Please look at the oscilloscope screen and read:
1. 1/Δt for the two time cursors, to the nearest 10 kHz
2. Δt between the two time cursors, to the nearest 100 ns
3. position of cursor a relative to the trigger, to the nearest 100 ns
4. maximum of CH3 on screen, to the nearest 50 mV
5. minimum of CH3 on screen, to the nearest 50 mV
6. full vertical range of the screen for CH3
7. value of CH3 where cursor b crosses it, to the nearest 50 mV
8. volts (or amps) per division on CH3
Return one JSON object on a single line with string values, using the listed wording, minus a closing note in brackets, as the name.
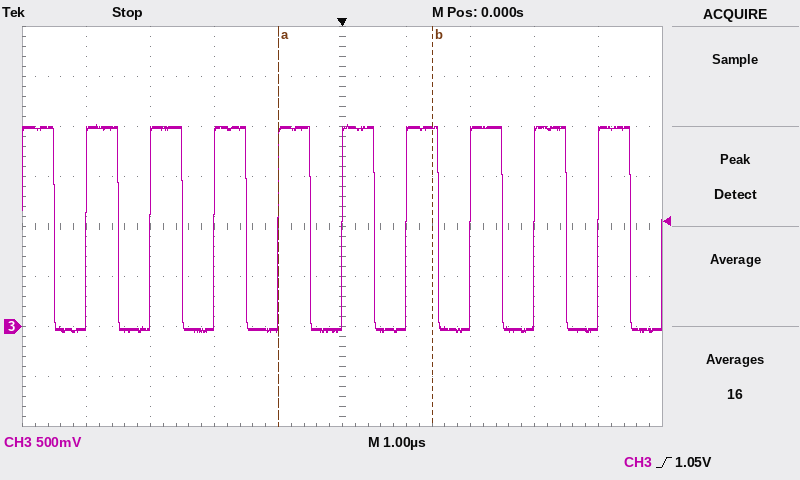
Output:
{"1/Δt for the two time cursors, to the nearest 10 kHz": "420 kHz", "Δt between the two time cursors, to the nearest 100 ns": "2.4 µs", "position of cursor a relative to the trigger, to the nearest 100 ns": "-1.0 µs", "maximum of CH3 on screen, to the nearest 50 mV": "2.00 V", "minimum of CH3 on screen, to the nearest 50 mV": "-50 mV", "full vertical range of the screen for CH3": "4 V", "value of CH3 where cursor b crosses it, to the nearest 50 mV": "2.00 V", "volts (or amps) per division on CH3": "500 mV"}
